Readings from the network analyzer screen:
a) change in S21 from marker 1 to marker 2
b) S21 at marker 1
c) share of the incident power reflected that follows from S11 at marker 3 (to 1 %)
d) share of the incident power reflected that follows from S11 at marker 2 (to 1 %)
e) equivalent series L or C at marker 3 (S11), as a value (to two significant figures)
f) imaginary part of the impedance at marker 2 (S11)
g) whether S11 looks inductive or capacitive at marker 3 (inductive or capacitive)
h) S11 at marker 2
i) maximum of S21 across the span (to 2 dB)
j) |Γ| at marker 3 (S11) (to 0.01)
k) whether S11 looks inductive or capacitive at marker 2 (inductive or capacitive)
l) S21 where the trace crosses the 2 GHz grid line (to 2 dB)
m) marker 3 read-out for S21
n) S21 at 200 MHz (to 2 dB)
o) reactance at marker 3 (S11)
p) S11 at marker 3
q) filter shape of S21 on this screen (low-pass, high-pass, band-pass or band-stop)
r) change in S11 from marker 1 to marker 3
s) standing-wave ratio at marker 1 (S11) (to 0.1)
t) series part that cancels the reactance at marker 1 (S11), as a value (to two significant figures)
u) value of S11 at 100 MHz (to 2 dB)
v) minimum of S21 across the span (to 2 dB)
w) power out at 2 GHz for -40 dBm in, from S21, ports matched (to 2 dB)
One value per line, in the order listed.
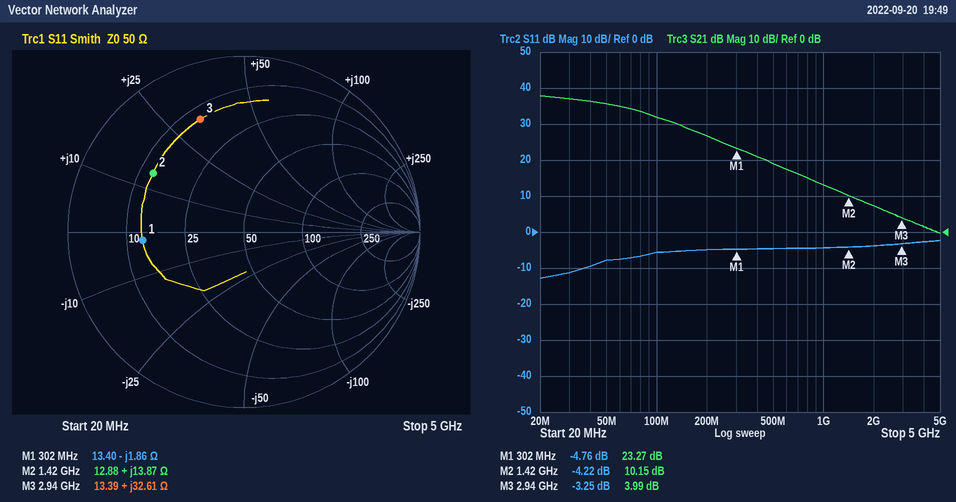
-13.12 dB
23.27 dB
47 %
38 %
1.8 nH
+13.87 Ω
inductive
-4.22 dB
38 dB
0.69
inductive
8 dB
3.99 dB
26 dB
+32.61 Ω
-3.25 dB
low-pass
1.51 dB
3.7
980 pH
-6 dB
0 dB
-32 dBm
